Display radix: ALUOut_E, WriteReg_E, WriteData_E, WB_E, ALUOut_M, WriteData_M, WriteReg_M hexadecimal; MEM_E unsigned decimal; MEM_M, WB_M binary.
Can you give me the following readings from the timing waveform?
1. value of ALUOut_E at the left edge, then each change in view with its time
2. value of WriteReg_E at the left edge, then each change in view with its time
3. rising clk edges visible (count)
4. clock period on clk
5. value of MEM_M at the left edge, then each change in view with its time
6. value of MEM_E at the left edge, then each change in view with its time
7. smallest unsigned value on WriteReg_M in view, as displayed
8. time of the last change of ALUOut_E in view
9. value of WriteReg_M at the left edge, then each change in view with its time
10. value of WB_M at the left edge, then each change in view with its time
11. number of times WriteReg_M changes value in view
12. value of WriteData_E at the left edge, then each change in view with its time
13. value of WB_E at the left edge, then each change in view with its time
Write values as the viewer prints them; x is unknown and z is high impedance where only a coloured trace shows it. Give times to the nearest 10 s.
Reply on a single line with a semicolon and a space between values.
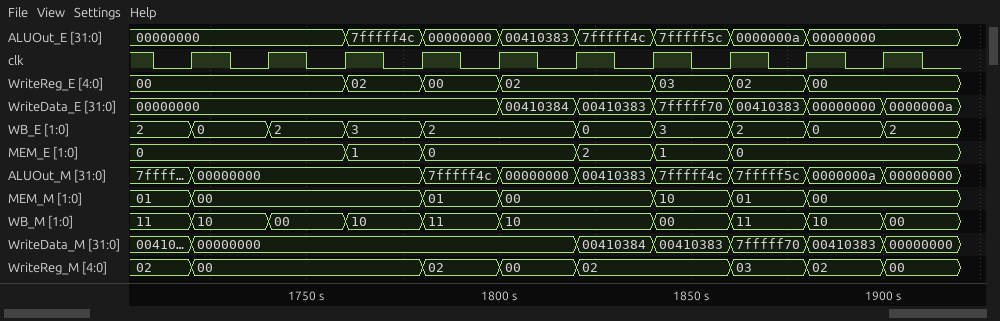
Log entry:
00000000, 7fffff4c at 1760 s, 00000000 at 1780 s, 00410383 at 1800 s, 7fffff4c at 1820 s, 7fffff5c at 1840 s, 0000000a at 1860 s, 00000000 at 1880 s; 00, 02 at 1760 s, 00 at 1780 s, 02 at 1800 s, 03 at 1840 s, 02 at 1860 s, 00 at 1880 s; 10; 20 s; 01, 00 at 1720 s, 01 at 1780 s, 00 at 1800 s, 10 at 1840 s, 01 at 1860 s, 00 at 1880 s; 0, 1 at 1760 s, 0 at 1780 s, 2 at 1820 s, 1 at 1840 s, 0 at 1860 s; 00; 1880 s; 02, 00 at 1720 s, 02 at 1780 s, 00 at 1800 s, 02 at 1820 s, 03 at 1860 s, 02 at 1880 s, 00 at 1900 s; 11, 10 at 1720 s, 00 at 1740 s, 10 at 1760 s, 11 at 1780 s, 10 at 1800 s, 00 at 1840 s, 11 at 1860 s, 10 at 1880 s, 00 at 1900 s; 7; 00000000, 00410384 at 1800 s, 00410383 at 1820 s, 7fffff70 at 1840 s, 00410383 at 1860 s, 00000000 at 1880 s, 0000000a at 1900 s; 2, 0 at 1720 s, 2 at 1740 s, 3 at 1760 s, 2 at 1780 s, 0 at 1820 s, 3 at 1840 s, 2 at 1860 s, 0 at 1880 s, 2 at 1900 s
